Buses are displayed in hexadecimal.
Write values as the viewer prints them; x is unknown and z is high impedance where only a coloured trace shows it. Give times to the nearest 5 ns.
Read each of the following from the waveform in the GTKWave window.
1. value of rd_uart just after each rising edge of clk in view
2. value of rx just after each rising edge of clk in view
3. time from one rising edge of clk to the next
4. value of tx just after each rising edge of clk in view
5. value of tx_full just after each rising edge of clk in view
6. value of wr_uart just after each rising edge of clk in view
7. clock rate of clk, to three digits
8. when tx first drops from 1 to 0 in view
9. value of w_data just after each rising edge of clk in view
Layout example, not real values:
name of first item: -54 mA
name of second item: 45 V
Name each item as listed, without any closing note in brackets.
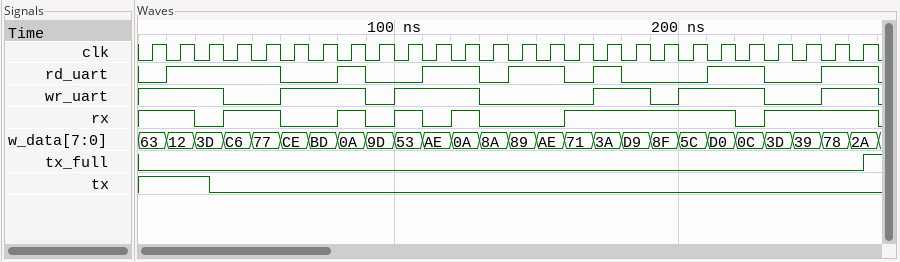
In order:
value of rd_uart just after each rising edge of clk in view: 0 1 1 1 1 0 0 1 0 0 1 1 0 1 1 0 1 0 0 0 1 1 0 0 1 1
value of rx just after each rising edge of clk in view: 1 1 0 1 1 0 0 1 0 1 0 1 0 0 0 1 1 1 1 1 1 0 1 1 1 1
time from one rising edge of clk to the next: 10 ns
value of tx just after each rising edge of clk in view: 1 1 0 0 0 0 0 0 0 0 0 0 0 0 0 0 0 0 0 0 0 0 0 0 0 0
value of tx_full just after each rising edge of clk in view: 0 0 0 0 0 0 0 0 0 0 0 0 0 0 0 0 0 0 0 0 0 0 0 0 0 1
value of wr_uart just after each rising edge of clk in view: 1 1 1 0 0 1 1 1 0 1 1 1 0 0 0 0 1 1 0 1 1 1 0 0 1 1
clock rate of clk, to three digits: 100 MHz
when tx first drops from 1 to 0 in view: 35 ns
value of w_data just after each rising edge of clk in view: 63, 12, 3D, C6, 77, CE, BD, 0A, 9D, 53, AE, 0A, 8A, 89, AE, 71, 3A, D9, 8F, 5C, D0, 0C, 3D, 39, 78, 2A
